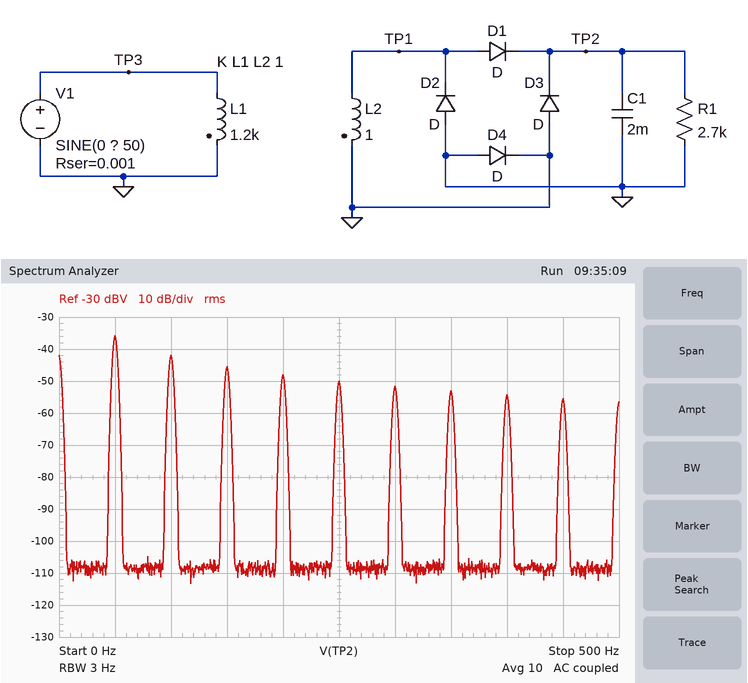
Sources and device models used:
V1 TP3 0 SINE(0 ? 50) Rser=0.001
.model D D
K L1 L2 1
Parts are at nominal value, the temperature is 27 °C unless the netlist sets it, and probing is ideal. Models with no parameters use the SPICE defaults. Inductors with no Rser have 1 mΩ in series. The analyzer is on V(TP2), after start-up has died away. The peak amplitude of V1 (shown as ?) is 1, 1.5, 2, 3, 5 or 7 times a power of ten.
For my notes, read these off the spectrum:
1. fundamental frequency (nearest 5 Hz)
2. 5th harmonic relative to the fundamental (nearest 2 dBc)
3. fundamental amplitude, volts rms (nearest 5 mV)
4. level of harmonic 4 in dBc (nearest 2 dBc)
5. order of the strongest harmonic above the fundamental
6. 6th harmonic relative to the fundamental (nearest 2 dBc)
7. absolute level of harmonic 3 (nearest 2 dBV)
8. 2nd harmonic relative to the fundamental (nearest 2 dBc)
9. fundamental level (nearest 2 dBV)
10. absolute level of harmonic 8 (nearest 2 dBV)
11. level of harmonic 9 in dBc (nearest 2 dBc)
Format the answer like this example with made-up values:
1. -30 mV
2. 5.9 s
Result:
1. 50 Hz
2. -14 dBc
3. 15 mV
4. -12 dBc
5. 2
6. -16 dBc
7. -46 dBV
8. -6 dBc
9. -36 dBV
10. -54 dBV
11. -20 dBc
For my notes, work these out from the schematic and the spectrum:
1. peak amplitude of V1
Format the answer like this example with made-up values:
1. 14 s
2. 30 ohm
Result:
1. 700 V
